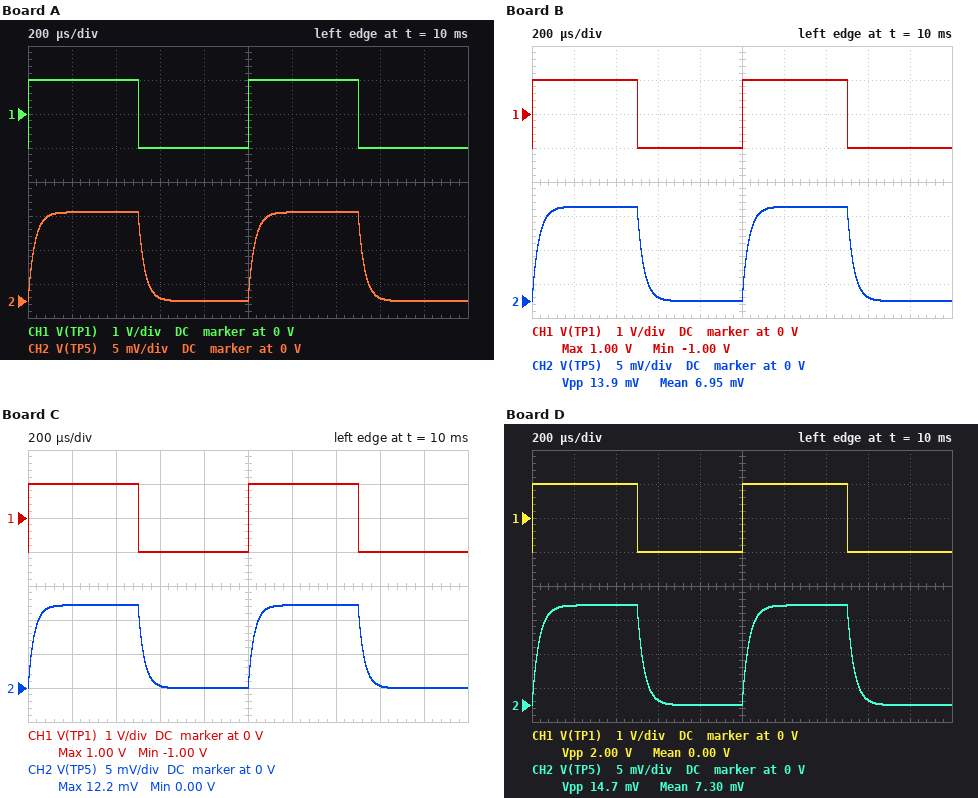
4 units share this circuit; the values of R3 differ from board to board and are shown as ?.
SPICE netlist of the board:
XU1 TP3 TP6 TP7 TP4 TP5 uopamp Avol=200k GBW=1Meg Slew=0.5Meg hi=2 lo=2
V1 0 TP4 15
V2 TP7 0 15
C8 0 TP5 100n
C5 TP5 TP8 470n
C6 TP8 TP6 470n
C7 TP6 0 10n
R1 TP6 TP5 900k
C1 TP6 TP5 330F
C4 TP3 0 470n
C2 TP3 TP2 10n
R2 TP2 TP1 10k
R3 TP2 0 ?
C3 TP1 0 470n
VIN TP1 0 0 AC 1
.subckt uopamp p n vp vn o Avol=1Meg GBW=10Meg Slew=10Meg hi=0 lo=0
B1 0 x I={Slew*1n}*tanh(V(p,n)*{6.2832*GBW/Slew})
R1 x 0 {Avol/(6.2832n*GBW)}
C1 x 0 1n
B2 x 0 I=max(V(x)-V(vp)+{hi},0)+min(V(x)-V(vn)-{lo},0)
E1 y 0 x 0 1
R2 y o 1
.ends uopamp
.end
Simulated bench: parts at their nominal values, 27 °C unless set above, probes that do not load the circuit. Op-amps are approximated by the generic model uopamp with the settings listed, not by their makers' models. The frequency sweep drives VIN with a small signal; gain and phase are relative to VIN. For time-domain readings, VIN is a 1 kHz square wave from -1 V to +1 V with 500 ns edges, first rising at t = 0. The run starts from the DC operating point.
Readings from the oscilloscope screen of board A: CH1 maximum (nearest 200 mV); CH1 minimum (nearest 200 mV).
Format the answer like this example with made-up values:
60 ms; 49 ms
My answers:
1.0 V; -1.0 V
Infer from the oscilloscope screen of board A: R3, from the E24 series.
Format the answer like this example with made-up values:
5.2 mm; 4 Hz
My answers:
4.3 kΩ
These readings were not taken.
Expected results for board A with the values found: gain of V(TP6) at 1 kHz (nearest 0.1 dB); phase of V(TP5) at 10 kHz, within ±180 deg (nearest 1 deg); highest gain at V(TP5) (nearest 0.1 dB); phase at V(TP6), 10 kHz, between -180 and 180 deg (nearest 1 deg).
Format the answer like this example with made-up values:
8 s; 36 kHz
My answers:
-44.2 dB; -62 deg; -43.7 dB; -62 deg
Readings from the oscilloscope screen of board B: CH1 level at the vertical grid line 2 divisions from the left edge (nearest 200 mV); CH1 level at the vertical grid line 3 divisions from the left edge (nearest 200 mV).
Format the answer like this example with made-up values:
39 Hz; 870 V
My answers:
1.0 V; -1.0 V
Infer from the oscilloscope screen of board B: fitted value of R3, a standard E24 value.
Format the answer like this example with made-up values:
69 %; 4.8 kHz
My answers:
4.7 kΩ
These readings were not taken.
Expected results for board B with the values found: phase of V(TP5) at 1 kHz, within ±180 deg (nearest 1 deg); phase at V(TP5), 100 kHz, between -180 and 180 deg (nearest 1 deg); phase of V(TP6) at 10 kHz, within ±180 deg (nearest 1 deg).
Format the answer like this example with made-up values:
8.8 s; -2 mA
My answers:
-11 deg; -93 deg; -64 deg
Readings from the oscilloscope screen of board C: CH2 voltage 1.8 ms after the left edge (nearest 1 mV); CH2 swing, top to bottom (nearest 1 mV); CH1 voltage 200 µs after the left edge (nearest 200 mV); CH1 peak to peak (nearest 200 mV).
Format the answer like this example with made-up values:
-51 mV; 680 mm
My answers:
0 V; 12 mV; 1.0 V; 2.0 V
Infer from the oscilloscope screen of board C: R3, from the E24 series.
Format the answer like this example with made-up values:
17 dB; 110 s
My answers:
3.9 kΩ
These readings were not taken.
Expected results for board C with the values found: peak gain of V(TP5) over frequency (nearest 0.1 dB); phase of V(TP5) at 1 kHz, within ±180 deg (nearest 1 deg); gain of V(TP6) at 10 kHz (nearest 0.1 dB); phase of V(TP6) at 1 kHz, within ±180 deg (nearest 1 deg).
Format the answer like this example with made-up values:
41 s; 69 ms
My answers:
-44.3 dB; -10 deg; -50.7 dB; -10 deg
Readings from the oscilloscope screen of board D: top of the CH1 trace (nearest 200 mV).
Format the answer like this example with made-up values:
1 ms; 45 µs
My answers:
1.0 V
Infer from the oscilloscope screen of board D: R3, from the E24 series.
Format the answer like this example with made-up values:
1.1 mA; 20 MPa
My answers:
5.1 kΩ
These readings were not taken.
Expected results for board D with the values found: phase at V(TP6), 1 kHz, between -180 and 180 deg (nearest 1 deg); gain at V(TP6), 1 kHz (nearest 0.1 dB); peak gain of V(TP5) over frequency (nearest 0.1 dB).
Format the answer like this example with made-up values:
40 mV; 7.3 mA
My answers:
-12 deg; -43.2 dB; -42.7 dB
